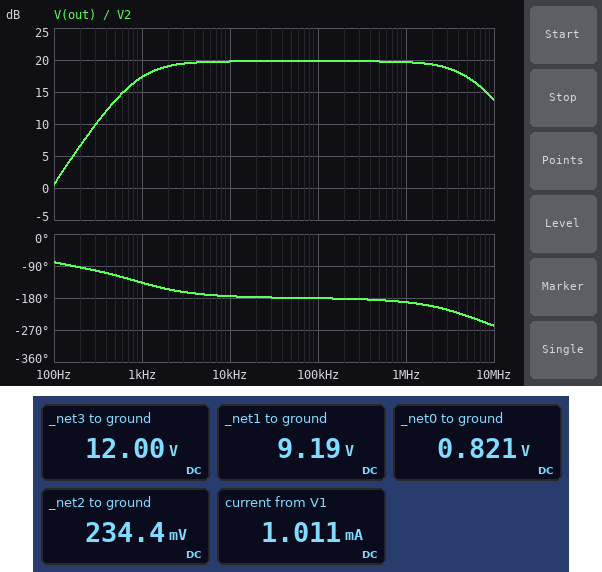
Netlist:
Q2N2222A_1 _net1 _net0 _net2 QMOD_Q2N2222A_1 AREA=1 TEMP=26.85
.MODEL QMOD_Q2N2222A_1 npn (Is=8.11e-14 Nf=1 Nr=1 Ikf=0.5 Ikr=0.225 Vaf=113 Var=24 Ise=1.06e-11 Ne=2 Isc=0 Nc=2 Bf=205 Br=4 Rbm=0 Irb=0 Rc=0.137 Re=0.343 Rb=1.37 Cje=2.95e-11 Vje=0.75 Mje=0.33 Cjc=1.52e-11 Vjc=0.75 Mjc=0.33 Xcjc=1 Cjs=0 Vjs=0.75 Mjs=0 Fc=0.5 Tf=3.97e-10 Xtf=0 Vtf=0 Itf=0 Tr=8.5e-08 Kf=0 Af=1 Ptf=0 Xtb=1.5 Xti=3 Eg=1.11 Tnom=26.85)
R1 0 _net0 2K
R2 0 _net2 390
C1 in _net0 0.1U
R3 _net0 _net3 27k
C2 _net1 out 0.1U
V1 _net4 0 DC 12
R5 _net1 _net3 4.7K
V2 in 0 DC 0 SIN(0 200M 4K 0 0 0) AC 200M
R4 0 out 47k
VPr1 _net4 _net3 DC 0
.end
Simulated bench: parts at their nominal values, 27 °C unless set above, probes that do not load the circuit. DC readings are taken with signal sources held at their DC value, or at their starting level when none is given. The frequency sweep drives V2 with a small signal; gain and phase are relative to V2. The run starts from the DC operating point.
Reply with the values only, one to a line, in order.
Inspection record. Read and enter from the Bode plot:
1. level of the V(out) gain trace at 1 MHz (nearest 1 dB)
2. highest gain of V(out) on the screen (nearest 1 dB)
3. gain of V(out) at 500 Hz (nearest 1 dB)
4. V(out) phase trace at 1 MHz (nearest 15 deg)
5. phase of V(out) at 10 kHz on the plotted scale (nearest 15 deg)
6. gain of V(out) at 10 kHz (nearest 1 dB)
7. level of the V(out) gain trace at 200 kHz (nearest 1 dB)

20 dB
20 dB
14 dB
-195 deg
-180 deg
20 dB
20 dB
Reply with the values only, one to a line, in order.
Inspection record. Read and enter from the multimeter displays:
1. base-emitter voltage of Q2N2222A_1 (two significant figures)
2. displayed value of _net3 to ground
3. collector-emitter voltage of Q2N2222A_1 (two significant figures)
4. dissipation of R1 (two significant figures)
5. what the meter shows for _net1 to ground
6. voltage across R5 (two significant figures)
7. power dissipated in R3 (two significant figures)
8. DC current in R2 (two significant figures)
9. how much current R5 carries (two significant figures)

590 mV
12.00 V
9.0 V
340 µW
9.19 V
2.8 V
4.6 mW
600 µA
600 µA
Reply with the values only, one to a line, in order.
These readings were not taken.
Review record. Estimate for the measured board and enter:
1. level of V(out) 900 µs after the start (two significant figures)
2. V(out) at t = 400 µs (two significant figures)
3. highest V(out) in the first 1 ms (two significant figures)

1.4 V
1.4 V
1.9 V
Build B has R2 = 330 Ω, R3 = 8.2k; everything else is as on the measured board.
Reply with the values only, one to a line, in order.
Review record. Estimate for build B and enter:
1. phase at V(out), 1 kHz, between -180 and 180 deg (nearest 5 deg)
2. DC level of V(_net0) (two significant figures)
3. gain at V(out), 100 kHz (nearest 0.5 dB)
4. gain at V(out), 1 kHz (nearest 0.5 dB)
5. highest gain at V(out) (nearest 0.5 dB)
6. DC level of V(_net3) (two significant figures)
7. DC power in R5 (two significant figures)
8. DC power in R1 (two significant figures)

80 deg
1.6 V
-1.5 dB
-17.0 dB
0 dB
12 V
26 mW
1.2 mW
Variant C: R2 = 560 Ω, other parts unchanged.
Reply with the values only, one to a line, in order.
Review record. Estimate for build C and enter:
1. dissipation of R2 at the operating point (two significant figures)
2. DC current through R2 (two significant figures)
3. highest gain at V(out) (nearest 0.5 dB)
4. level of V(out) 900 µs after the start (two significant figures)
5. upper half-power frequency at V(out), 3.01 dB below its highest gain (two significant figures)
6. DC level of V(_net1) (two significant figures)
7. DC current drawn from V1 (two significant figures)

110 µW
440 µA
16.5 dB
970 mV
6.0 MHz
10 V
850 µA
